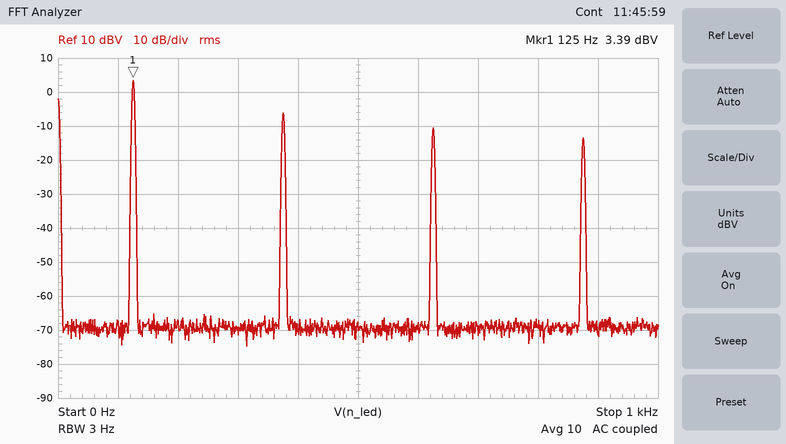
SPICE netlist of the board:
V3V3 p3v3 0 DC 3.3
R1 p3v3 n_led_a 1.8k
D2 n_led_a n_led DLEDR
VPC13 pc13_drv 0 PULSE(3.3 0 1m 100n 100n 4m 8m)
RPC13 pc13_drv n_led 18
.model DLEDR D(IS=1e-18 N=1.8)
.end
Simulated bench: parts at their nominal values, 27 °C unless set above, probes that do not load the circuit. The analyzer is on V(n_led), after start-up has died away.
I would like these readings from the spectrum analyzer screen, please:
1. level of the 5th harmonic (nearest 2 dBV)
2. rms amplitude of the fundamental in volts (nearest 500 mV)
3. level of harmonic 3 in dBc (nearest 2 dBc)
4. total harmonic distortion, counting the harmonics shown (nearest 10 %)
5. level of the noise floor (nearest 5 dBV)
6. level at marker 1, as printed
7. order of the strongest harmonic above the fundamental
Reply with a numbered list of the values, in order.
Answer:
1. -10 dBV
2. 1.5 V
3. -10 dBc
4. 40 %
5. -70 dBV
6. 3.39 dBV
7. 3
